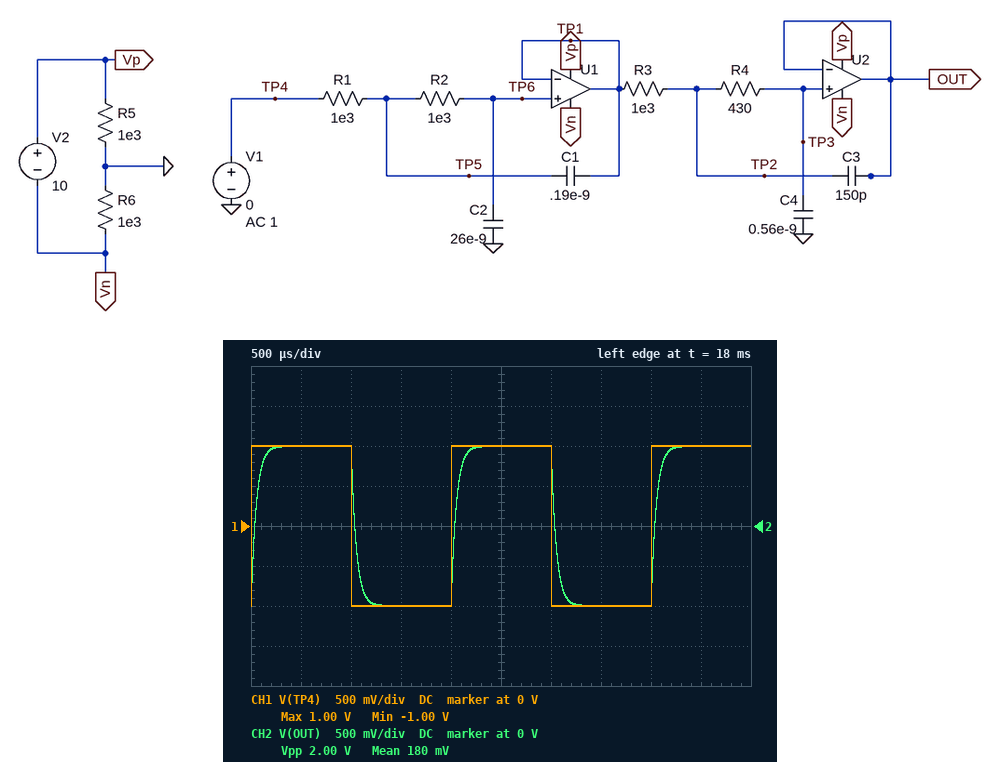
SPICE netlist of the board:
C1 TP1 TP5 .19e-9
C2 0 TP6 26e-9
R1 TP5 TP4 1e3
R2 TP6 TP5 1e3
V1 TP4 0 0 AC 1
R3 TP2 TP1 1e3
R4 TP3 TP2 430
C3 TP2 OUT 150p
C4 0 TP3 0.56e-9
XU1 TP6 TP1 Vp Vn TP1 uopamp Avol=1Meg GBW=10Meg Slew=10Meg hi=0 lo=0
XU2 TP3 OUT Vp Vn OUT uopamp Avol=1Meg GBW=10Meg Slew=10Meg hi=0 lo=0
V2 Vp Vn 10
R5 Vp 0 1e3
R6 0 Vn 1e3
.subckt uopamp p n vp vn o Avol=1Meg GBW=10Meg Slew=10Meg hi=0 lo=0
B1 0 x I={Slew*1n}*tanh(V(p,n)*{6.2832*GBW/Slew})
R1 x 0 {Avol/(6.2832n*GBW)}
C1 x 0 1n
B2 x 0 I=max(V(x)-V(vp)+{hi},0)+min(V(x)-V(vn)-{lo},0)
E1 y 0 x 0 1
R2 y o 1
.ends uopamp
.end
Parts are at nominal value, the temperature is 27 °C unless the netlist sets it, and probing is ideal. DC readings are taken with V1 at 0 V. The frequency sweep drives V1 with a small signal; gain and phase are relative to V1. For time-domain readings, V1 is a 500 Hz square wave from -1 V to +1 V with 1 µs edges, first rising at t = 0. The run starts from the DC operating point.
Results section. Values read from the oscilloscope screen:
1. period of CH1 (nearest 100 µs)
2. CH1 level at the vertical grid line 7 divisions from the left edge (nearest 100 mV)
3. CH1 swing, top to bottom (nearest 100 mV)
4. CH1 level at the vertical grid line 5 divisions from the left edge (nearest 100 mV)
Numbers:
2.0 ms
-1.0 V
2.0 V
1.0 V
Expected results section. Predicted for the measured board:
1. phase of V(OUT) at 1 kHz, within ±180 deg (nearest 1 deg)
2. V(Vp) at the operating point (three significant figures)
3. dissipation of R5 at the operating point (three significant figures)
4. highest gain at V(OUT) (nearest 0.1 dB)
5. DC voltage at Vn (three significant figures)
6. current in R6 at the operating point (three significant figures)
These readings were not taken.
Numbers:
-18 deg
5.00 V
25.0 mW
0 dB
-5.00 V
5.00 mA
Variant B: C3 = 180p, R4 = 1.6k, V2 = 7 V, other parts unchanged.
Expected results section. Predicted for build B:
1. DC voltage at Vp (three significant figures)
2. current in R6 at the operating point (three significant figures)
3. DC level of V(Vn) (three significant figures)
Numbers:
3.50 V
3.50 mA
-3.50 V
